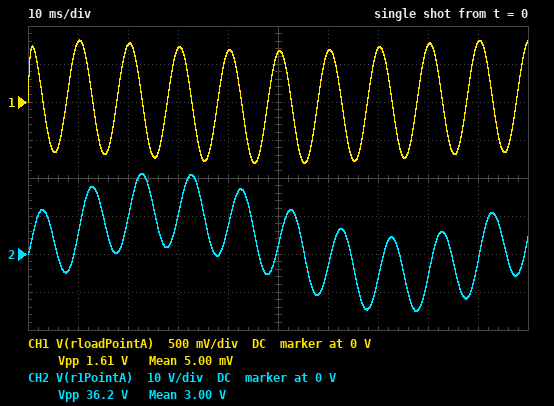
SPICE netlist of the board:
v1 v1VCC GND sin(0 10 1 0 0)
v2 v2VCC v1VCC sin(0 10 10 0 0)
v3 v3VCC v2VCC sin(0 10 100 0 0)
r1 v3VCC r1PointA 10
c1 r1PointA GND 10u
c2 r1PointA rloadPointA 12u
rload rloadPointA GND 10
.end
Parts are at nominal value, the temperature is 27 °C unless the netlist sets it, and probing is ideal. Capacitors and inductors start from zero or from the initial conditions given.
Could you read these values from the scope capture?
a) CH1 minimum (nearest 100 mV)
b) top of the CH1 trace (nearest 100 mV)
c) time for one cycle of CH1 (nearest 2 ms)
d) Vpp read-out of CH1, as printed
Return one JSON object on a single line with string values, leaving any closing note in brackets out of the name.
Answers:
{"CH1 minimum": "-800 mV", "top of the CH1 trace": "800 mV", "time for one cycle of CH1": "10 ms", "Vpp read-out of CH1, as printed": "1.61 V"}
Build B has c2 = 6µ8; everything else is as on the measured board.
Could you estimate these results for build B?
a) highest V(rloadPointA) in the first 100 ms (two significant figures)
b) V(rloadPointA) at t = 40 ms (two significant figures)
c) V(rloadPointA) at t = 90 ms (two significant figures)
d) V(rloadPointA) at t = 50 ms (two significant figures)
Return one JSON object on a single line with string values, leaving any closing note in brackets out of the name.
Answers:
{"highest V(rloadPointA) in the first 100 ms": "470 mV", "V(rloadPointA) at t = 40 ms": "390 mV", "V(rloadPointA) at t = 90 ms": "460 mV", "V(rloadPointA) at t = 50 ms": "380 mV"}
